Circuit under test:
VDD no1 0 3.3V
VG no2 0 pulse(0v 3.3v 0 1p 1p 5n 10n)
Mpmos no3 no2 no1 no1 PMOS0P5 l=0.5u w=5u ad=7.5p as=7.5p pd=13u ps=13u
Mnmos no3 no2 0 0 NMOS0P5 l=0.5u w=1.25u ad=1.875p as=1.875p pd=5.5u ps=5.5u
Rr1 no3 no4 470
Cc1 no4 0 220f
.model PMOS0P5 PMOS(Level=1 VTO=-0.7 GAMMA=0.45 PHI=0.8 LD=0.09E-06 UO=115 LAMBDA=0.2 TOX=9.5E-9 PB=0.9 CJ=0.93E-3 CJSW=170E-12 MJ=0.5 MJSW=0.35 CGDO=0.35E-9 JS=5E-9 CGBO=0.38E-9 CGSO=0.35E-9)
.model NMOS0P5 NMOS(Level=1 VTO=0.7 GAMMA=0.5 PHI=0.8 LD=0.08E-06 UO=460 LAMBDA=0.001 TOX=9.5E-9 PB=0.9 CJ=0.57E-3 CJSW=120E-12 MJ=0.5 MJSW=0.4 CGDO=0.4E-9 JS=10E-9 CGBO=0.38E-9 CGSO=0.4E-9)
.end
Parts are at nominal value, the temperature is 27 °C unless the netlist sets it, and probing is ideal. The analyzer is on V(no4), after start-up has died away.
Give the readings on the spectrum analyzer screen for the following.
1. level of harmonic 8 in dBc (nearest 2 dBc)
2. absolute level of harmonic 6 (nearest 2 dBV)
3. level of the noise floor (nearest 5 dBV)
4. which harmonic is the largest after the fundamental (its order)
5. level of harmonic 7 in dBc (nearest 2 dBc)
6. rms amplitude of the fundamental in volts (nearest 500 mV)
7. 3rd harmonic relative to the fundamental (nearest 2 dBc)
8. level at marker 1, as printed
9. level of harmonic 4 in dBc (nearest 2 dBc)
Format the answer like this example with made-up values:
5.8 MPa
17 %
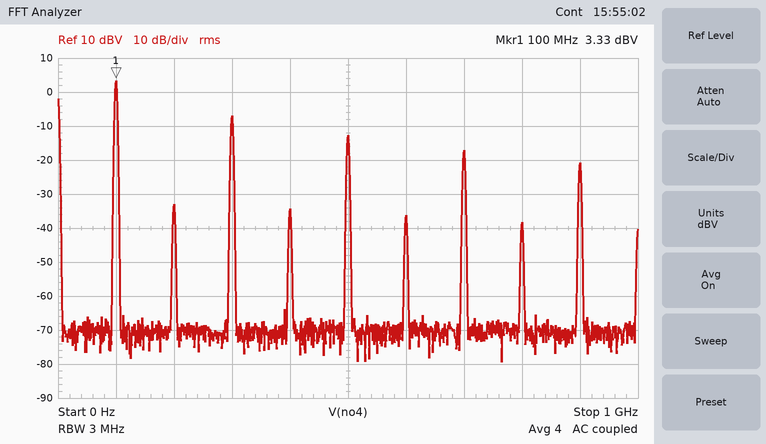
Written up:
-42 dBc
-36 dBV
-70 dBV
3
-20 dBc
1.5 V
-10 dBc
3.33 dBV
-38 dBc
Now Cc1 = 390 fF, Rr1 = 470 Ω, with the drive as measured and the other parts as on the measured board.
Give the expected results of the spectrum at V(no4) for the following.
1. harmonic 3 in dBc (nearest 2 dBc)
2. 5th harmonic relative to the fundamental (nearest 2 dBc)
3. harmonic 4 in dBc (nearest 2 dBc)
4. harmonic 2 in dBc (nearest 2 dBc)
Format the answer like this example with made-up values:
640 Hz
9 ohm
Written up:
-12 dBc
-18 dBc
-36 dBc
-32 dBc
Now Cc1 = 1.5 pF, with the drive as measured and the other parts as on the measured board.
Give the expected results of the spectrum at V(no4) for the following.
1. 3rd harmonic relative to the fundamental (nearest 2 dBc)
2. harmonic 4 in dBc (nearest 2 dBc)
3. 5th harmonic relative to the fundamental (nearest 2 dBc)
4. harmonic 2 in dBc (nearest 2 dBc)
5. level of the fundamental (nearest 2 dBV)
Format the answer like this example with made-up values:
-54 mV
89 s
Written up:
-18 dBc
-40 dBc
-26 dBc
-30 dBc
0 dBV
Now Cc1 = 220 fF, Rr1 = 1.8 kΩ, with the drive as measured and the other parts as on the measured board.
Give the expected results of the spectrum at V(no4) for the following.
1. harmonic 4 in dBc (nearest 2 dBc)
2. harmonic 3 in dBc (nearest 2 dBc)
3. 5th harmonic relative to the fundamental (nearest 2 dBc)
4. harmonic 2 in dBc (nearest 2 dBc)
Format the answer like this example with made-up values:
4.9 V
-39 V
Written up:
-46 dBc
-12 dBc
-20 dBc
-42 dBc
